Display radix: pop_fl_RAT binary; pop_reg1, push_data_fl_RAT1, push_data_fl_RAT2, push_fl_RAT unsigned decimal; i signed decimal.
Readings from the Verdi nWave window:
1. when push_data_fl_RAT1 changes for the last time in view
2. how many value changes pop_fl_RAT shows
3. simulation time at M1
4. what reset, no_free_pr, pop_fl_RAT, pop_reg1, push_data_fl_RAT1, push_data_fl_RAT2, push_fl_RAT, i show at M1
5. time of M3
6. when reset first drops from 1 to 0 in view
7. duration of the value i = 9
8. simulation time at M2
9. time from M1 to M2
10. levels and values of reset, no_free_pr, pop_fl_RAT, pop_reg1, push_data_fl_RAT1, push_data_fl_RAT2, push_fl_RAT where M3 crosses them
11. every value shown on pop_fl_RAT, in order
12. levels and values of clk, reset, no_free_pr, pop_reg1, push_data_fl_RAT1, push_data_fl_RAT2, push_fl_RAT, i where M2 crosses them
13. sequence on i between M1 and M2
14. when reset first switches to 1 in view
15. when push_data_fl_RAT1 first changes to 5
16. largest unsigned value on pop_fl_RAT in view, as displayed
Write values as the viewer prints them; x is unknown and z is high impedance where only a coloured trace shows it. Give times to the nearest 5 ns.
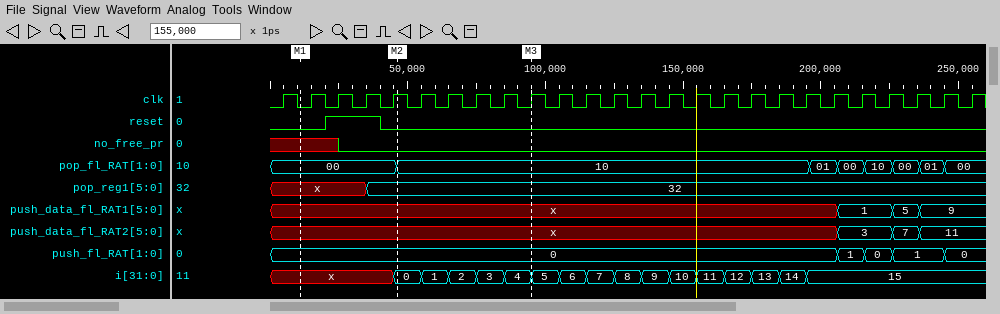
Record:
235 ns
7
10 ns
reset=0, no_free_pr=x, pop_fl_RAT=00, pop_reg1=x, push_data_fl_RAT1=x, push_data_fl_RAT2=x, push_fl_RAT=0, i=x
95 ns
40 ns
10 ns
45 ns
35 ns
reset=0, no_free_pr=0, pop_fl_RAT=10, pop_reg1=32, push_data_fl_RAT1=x, push_data_fl_RAT2=x, push_fl_RAT=0
00, 10, 01, 00, 10, 00, 01, 00
clk=1, reset=0, no_free_pr=0, pop_reg1=32, push_data_fl_RAT1=x, push_data_fl_RAT2=x, push_fl_RAT=0, i=0
x, 0
20 ns
225 ns
10
